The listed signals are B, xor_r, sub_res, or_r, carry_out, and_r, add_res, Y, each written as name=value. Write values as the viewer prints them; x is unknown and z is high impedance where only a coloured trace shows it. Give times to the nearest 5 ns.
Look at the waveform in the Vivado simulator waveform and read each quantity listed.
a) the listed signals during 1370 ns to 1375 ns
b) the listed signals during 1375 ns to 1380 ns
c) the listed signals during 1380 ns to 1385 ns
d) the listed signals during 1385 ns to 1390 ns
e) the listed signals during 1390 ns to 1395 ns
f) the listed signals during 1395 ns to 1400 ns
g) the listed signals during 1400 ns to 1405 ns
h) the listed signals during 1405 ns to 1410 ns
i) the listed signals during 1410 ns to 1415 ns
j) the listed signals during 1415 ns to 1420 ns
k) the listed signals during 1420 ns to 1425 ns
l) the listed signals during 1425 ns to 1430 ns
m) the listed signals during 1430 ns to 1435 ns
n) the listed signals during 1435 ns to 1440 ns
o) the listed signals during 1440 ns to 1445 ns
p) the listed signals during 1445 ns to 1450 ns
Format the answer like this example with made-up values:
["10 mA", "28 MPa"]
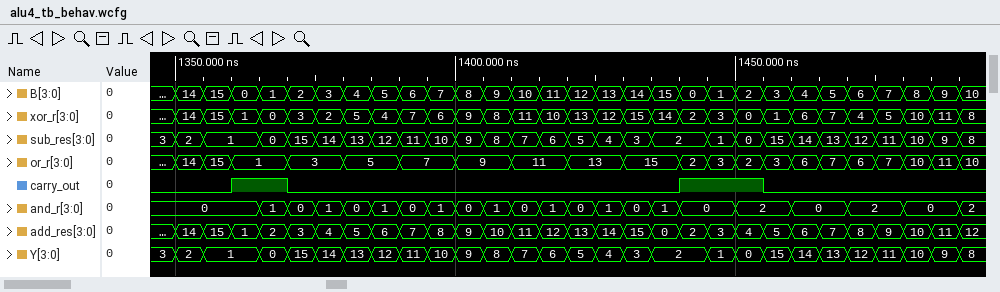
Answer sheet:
["B=2, xor_r=3, sub_res=15, or_r=3, carry_out=0, and_r=0, add_res=3, Y=15", "B=3, xor_r=2, sub_res=14, or_r=3, carry_out=0, and_r=1, add_res=4, Y=14", "B=4, xor_r=5, sub_res=13, or_r=5, carry_out=0, and_r=0, add_res=5, Y=13", "B=5, xor_r=4, sub_res=12, or_r=5, carry_out=0, and_r=1, add_res=6, Y=12", "B=6, xor_r=7, sub_res=11, or_r=7, carry_out=0, and_r=0, add_res=7, Y=11", "B=7, xor_r=6, sub_res=10, or_r=7, carry_out=0, and_r=1, add_res=8, Y=10", "B=8, xor_r=9, sub_res=9, or_r=9, carry_out=0, and_r=0, add_res=9, Y=9", "B=9, xor_r=8, sub_res=8, or_r=9, carry_out=0, and_r=1, add_res=10, Y=8", "B=10, xor_r=11, sub_res=7, or_r=11, carry_out=0, and_r=0, add_res=11, Y=7", "B=11, xor_r=10, sub_res=6, or_r=11, carry_out=0, and_r=1, add_res=12, Y=6", "B=12, xor_r=13, sub_res=5, or_r=13, carry_out=0, and_r=0, add_res=13, Y=5", "B=13, xor_r=12, sub_res=4, or_r=13, carry_out=0, and_r=1, add_res=14, Y=4", "B=14, xor_r=15, sub_res=3, or_r=15, carry_out=0, and_r=0, add_res=15, Y=3", "B=15, xor_r=14, sub_res=2, or_r=15, carry_out=0, and_r=1, add_res=0, Y=2", "B=0, xor_r=2, sub_res=2, or_r=2, carry_out=1, and_r=0, add_res=2, Y=2", "B=1, xor_r=3, sub_res=1, or_r=3, carry_out=1, and_r=0, add_res=3, Y=1"]
